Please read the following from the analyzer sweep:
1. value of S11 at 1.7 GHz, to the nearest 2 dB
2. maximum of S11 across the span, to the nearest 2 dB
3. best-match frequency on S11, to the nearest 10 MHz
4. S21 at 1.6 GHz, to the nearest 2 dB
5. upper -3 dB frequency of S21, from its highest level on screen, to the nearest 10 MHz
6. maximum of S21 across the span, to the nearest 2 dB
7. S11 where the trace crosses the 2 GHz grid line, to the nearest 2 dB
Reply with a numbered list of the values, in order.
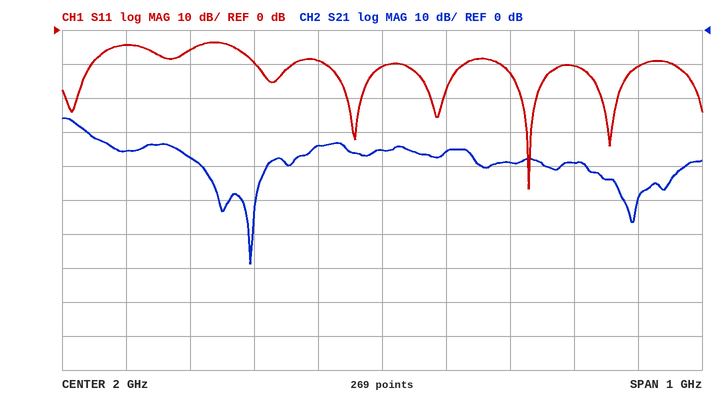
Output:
1. -6 dB
2. -4 dB
3. 2.23 GHz
4. -36 dB
5. 1.53 GHz
6. -26 dB
7. -10 dB
